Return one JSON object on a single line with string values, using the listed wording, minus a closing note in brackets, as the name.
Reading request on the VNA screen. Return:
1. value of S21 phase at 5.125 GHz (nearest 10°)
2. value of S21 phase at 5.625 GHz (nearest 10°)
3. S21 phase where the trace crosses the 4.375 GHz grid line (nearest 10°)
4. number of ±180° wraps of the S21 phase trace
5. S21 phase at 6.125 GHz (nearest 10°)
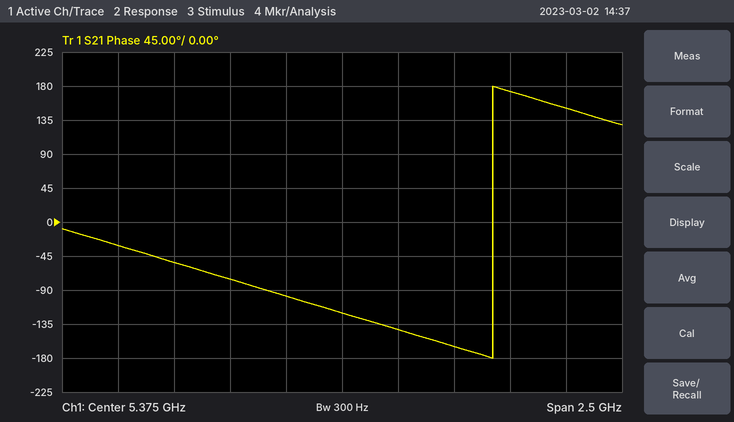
{"value of S21 phase at 5.125 GHz": "-100°", "value of S21 phase at 5.625 GHz": "-140°", "S21 phase where the trace crosses the 4.375 GHz grid line": "-30°", "number of ±180° wraps of the S21 phase trace": "1", "S21 phase at 6.125 GHz": "170°"}
